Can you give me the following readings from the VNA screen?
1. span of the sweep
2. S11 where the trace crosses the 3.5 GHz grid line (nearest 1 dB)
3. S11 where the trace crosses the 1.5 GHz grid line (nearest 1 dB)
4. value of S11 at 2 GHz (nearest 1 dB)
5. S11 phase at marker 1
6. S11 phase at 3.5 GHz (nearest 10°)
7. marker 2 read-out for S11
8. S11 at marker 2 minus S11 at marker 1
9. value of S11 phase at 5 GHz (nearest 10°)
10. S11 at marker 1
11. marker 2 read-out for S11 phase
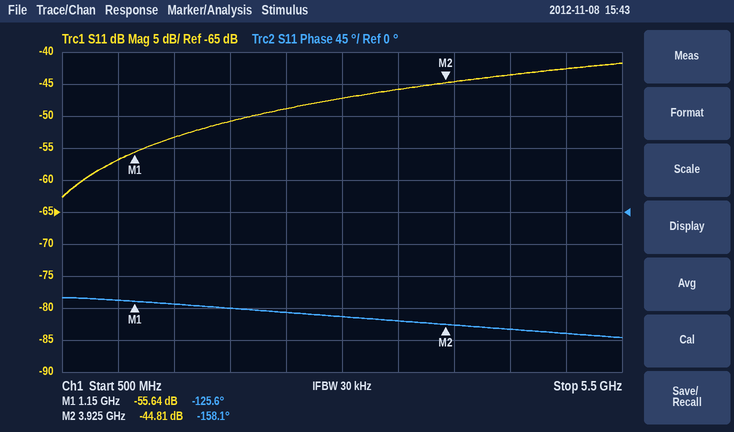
5 GHz
-46 dB
-53 dB
-51 dB
-125.6°
-150°
-44.81 dB
10.83 dB
-170°
-55.64 dB
-158.1°
